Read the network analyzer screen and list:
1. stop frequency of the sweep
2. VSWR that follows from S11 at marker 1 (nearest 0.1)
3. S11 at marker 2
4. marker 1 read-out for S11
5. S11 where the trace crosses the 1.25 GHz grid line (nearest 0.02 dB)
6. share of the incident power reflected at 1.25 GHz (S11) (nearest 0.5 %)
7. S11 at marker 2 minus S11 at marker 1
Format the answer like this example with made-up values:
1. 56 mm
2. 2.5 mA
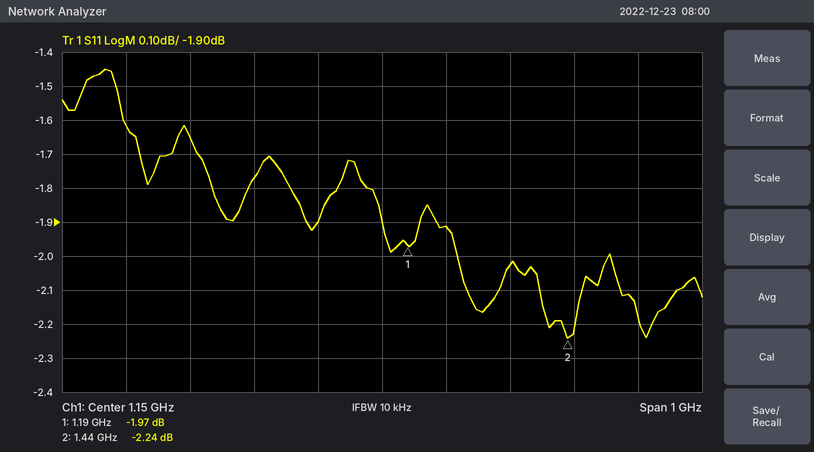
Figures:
1. 1.65 GHz
2. 8.9
3. -2.24 dB
4. -1.97 dB
5. -1.92 dB
6. 64.5 %
7. -0.27 dB
